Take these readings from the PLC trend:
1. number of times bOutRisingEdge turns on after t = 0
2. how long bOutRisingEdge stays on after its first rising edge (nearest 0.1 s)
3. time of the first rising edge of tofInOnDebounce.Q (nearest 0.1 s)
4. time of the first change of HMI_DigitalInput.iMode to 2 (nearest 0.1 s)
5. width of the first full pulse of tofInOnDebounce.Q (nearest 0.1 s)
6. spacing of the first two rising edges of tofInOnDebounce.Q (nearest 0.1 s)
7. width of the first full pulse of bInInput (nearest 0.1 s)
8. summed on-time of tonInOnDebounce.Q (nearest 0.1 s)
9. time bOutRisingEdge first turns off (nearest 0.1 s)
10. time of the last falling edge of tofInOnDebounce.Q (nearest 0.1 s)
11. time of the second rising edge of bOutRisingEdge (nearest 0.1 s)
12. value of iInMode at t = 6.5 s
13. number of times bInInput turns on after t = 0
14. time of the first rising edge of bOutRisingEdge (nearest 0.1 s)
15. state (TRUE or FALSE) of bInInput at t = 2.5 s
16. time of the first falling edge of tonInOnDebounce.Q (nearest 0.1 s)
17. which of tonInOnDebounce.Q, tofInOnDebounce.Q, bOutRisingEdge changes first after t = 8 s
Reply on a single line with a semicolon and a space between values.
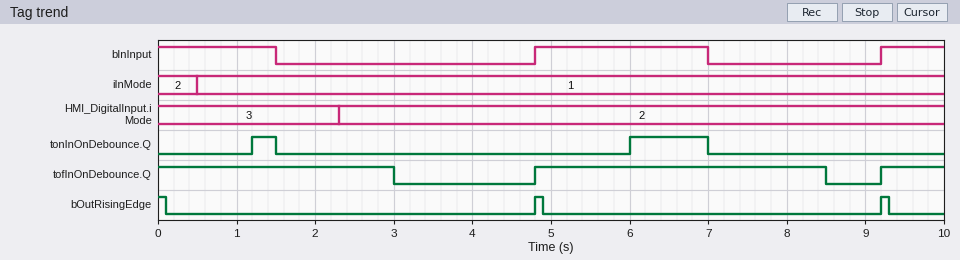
2; 0.1 s; 4.8 s; 2.3 s; 3.7 s; 4.4 s; 2.2 s; 1.3 s; 0.1 s; 8.5 s; 9.2 s; 1; 2; 4.8 s; FALSE; 1.5 s; tofInOnDebounce.Q
